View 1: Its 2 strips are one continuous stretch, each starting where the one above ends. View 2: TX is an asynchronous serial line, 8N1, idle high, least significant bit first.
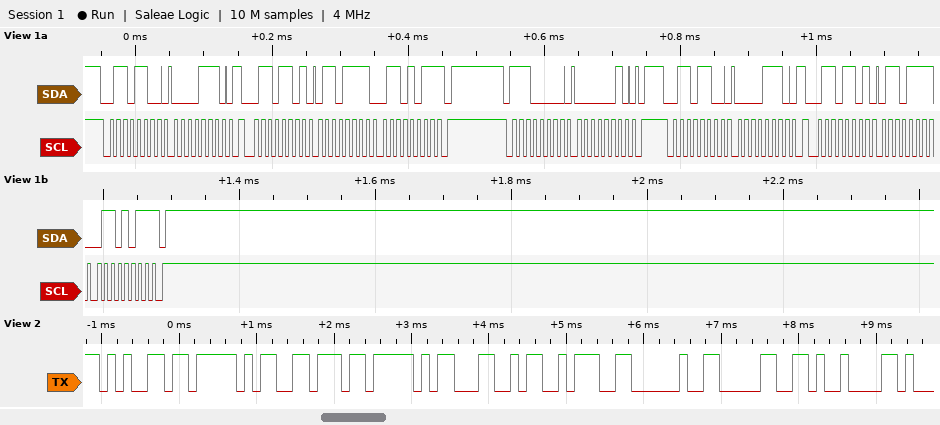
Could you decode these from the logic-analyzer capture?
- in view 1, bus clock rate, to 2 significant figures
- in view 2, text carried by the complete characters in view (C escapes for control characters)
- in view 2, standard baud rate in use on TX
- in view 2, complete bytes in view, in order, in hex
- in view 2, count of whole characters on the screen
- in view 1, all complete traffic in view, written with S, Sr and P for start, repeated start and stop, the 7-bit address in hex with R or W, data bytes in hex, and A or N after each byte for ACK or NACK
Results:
100 kHz
"e_v_L: 0\t"
9600 baud
65 5F 76 5F 4C 3A 20 30 09
9
S 36W A 0E A Sr 36R A 6F A 6B N P S 70W A 02 A P S 36W A 0E A Sr 36R A 6F A 6B N P
